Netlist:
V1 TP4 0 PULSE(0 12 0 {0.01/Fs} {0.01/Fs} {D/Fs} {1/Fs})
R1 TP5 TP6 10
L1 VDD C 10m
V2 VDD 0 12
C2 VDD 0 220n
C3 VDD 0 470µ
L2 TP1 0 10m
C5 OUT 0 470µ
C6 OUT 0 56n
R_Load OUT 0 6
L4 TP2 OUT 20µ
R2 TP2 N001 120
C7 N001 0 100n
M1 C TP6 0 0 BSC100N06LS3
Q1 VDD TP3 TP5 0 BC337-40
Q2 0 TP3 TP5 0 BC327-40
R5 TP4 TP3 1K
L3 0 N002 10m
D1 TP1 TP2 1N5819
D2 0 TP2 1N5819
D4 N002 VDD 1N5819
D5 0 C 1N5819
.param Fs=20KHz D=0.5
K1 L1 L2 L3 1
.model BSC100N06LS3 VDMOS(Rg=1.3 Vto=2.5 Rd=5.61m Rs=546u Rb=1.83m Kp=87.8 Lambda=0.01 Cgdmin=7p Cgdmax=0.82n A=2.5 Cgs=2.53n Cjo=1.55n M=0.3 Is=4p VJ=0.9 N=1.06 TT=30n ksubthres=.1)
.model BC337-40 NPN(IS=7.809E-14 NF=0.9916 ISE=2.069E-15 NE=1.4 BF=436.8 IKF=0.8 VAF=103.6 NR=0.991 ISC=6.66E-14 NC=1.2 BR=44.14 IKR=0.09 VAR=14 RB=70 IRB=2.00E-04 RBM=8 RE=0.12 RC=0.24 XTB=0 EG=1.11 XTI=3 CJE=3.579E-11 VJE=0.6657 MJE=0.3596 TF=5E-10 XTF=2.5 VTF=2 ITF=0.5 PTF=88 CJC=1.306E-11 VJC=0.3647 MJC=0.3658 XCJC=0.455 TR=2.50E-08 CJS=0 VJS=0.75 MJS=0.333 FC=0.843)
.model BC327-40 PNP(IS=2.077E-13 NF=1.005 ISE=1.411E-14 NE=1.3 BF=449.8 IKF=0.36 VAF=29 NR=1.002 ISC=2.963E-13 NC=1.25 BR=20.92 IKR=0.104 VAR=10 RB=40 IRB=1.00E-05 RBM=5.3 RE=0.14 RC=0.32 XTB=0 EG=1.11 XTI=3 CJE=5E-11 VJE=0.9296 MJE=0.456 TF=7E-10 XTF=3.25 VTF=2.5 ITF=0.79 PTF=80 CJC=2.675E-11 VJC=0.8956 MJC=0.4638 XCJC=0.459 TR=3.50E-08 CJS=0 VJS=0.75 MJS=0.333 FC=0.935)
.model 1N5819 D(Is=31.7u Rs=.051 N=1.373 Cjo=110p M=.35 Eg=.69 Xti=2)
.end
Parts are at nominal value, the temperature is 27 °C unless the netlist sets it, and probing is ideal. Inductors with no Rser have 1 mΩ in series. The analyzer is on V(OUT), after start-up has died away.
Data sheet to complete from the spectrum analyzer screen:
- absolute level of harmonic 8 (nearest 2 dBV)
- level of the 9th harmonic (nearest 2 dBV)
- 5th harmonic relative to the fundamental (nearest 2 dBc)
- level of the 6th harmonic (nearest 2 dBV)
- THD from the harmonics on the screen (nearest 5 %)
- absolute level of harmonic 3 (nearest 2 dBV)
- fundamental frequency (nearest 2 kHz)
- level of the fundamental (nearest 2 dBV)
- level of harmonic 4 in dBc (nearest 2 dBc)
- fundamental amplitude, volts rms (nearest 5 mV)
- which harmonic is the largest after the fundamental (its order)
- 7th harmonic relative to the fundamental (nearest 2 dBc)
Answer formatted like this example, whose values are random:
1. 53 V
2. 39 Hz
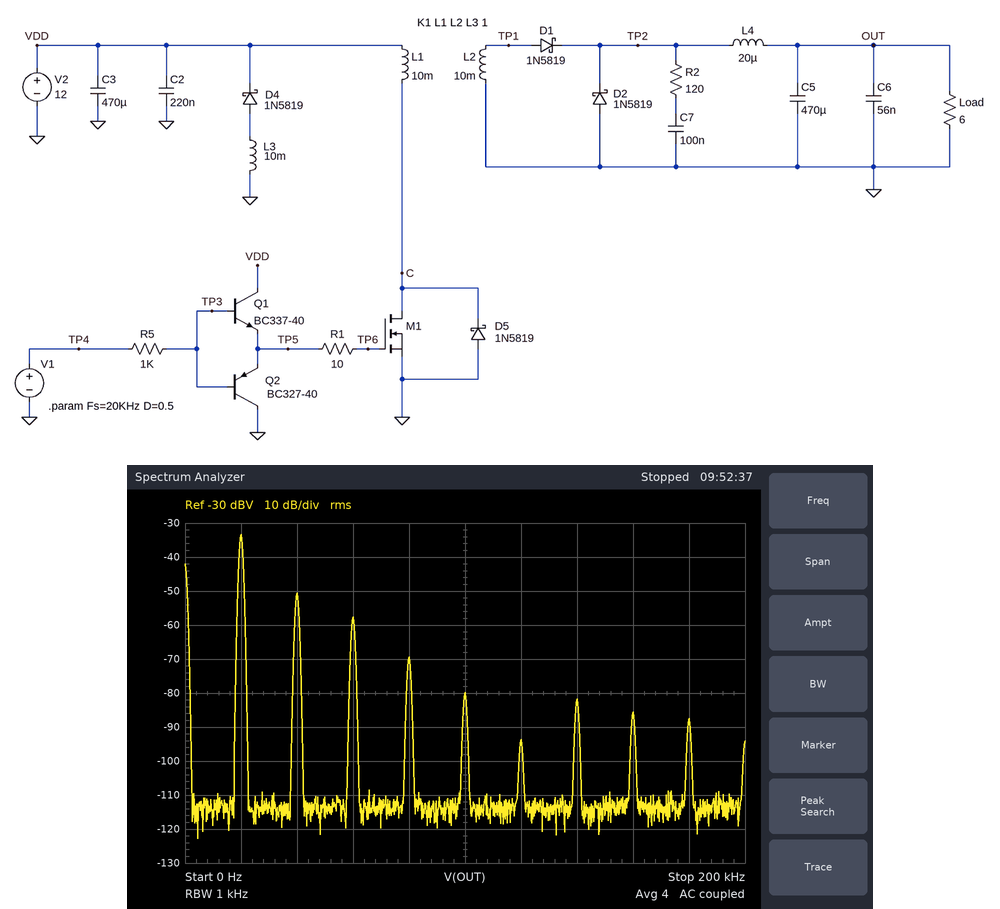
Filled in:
1. -86 dBV
2. -88 dBV
3. -46 dBc
4. -94 dBV
5. 15 %
6. -58 dBV
7. 20 kHz
8. -34 dBV
9. -36 dBc
10. 20 mV
11. 2
12. -48 dBc
